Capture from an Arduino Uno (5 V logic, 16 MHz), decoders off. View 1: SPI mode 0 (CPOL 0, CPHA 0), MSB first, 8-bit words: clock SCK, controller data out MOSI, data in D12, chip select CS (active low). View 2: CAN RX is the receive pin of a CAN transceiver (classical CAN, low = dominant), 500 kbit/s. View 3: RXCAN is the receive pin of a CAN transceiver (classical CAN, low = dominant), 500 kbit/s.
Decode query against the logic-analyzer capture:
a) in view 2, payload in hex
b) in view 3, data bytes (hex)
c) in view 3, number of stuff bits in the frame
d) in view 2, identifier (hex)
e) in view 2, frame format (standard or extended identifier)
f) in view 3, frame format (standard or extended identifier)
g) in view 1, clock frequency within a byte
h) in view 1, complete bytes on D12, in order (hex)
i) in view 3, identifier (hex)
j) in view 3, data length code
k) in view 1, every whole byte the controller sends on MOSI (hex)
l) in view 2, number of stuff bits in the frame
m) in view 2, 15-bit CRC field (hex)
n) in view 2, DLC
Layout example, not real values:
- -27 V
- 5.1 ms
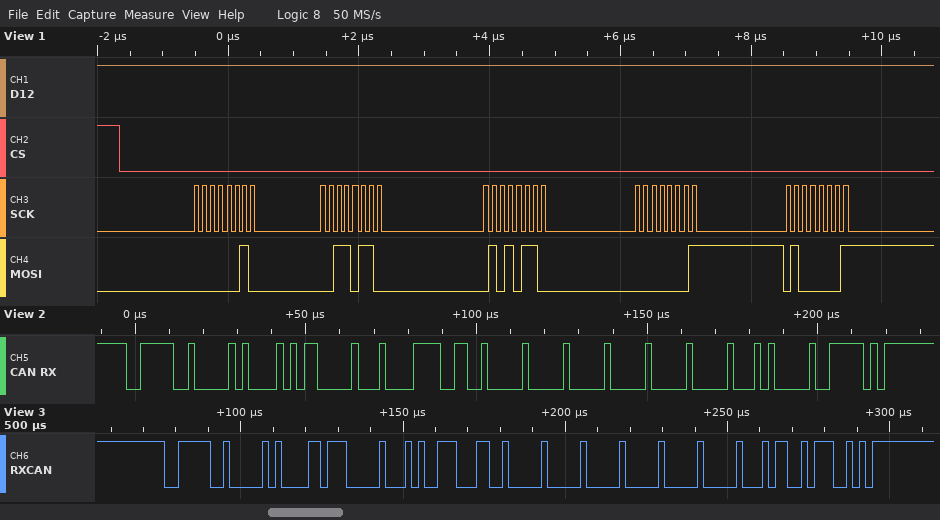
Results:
- 56 01 0F 32 00 00 00 00
- 6E 01 4E 32 00 00 00 00
- 9
- 0x3E8
- standard
- standard
- 8 MHz
- FF FF FF FF FF
- 0x3E8
- 8
- 02 36 56 01 41
- 11
- 0x501F
- 8
